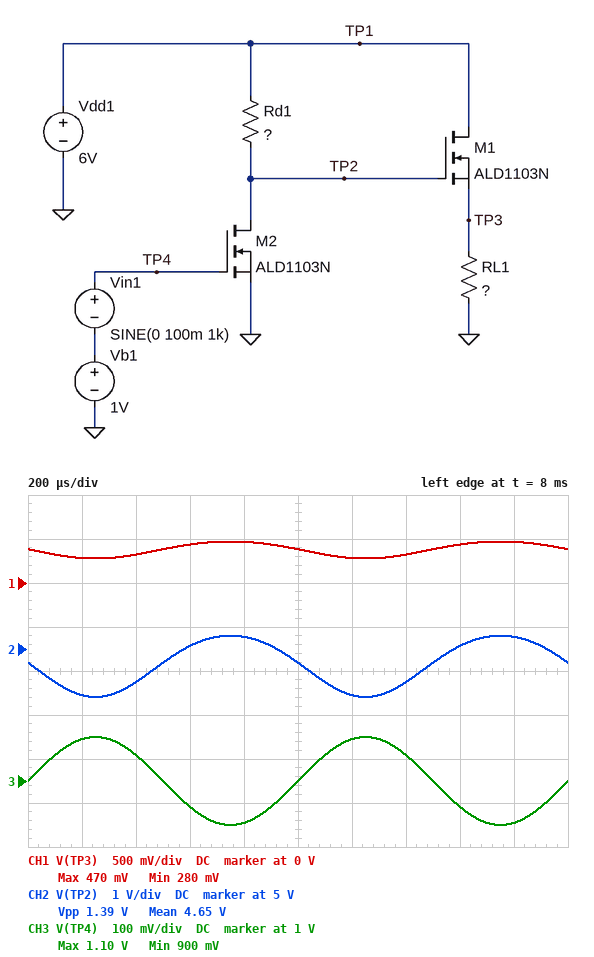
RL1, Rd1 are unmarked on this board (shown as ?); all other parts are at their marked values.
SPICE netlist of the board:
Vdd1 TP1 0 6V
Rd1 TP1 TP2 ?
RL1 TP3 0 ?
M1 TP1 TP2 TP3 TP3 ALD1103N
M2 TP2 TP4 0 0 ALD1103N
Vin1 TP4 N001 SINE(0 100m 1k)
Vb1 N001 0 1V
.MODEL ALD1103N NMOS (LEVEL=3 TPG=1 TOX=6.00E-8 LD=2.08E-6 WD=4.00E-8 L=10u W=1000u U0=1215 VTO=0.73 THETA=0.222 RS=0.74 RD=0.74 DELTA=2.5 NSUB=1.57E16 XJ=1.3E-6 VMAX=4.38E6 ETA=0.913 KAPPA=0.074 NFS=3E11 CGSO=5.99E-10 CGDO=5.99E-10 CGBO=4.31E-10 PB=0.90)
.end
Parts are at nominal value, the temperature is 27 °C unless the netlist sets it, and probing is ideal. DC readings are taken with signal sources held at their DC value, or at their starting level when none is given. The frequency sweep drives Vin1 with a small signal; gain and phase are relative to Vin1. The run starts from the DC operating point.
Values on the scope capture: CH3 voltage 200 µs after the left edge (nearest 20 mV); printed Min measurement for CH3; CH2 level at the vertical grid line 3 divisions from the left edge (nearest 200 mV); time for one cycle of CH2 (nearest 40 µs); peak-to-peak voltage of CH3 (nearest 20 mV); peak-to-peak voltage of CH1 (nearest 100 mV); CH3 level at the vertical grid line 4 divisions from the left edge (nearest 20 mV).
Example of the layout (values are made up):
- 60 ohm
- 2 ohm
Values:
- 1.10 V
- 900 mV
- 5.0 V
- 1.00 ms
- 200 mV
- 200 mV
- 900 mV
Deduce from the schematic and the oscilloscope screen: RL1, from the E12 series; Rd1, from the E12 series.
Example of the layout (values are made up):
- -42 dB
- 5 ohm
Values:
- 12 Ω
- 2.7 kΩ
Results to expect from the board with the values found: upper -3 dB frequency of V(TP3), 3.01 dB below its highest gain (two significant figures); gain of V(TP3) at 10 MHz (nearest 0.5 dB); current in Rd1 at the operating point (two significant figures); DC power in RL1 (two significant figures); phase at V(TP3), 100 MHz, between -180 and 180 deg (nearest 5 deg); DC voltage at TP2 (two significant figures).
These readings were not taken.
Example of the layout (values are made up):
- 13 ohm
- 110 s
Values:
- 17 MHz
- -1.5 dB
- 490 µA
- 12 mW
- 100 deg
- 4.7 V
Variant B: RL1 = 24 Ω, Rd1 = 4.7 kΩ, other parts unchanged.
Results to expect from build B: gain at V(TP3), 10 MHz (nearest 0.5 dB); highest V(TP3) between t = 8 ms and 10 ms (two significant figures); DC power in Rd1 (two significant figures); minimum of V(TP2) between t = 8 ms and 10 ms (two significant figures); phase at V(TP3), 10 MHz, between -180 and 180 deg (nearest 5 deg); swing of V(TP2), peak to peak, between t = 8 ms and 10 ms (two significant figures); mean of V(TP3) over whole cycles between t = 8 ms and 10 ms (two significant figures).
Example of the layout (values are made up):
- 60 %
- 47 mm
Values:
- 5.5 dB
- 700 mV
- 1.0 mW
- 2.5 V
- 135 deg
- 2.3 V
- 460 mV
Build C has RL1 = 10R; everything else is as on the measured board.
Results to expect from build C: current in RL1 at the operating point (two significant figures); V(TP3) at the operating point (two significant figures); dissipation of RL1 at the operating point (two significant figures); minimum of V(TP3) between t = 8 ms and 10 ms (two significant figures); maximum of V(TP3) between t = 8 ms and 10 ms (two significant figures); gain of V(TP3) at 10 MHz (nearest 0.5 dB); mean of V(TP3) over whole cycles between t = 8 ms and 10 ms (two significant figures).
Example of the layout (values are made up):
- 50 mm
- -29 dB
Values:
- 33 mA
- 330 mV
- 11 mW
- 240 mV
- 400 mV
- -3.0 dB
- 320 mV
